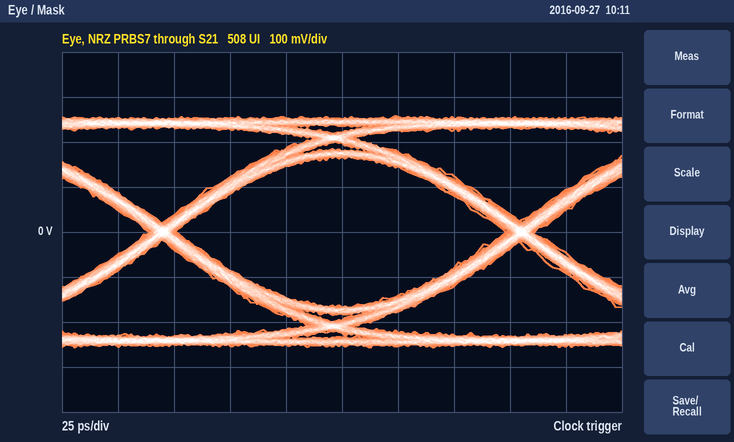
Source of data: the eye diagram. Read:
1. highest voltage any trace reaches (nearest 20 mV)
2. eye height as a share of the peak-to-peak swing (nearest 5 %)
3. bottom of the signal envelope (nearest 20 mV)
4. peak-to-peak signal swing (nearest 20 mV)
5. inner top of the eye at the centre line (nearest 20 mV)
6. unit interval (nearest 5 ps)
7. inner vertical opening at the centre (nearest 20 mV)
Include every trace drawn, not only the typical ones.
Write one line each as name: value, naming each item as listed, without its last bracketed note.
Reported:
highest voltage any trace reaches: 260 mV
eye height as a share of the peak-to-peak swing: 65 %
bottom of the signal envelope: -260 mV
peak-to-peak signal swing: 520 mV
inner top of the eye at the centre line: 160 mV
unit interval: 160 ps
inner vertical opening at the centre: 340 mV
